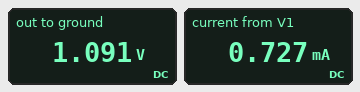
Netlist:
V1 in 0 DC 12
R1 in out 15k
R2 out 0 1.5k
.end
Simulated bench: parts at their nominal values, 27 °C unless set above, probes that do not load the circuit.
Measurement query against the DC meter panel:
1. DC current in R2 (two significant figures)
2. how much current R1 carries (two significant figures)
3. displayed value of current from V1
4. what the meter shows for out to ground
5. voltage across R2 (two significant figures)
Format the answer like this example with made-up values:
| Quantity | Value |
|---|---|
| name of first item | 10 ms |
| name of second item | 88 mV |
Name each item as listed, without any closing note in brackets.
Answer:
| Quantity | Value |
|---|---|
| DC current in R2 | 730 µA |
| how much current R1 carries | 730 µA |
| displayed value of current from V1 | 0.727 mA |
| what the meter shows for out to ground | 1.091 V |
| voltage across R2 | 1.1 V |
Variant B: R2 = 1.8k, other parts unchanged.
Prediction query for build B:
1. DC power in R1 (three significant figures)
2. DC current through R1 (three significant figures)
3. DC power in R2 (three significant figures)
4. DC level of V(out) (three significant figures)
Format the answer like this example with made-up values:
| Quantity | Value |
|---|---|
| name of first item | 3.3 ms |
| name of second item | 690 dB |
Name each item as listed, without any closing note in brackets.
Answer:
| Quantity | Value |
|---|---|
| DC power in R1 | 7.65 mW |
| DC current through R1 | 714 µA |
| DC power in R2 | 918 µW |
| DC level of V(out) | 1.29 V |
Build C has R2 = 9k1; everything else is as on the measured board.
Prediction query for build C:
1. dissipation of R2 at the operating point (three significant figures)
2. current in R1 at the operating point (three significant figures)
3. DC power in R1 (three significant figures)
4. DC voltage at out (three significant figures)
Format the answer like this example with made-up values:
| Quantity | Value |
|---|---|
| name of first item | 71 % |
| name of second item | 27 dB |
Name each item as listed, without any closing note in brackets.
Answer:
| Quantity | Value |
|---|---|
| dissipation of R2 at the operating point | 2.26 mW |
| current in R1 at the operating point | 498 µA |
| DC power in R1 | 3.72 mW |
| DC voltage at out | 4.53 V |
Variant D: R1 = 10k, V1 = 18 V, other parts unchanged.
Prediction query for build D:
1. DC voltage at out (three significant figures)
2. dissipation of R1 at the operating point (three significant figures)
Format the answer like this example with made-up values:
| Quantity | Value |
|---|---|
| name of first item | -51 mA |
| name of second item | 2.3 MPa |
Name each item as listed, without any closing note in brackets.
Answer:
| Quantity | Value |
|---|---|
| DC voltage at out | 2.35 V |
| dissipation of R1 at the operating point | 24.5 mW |
